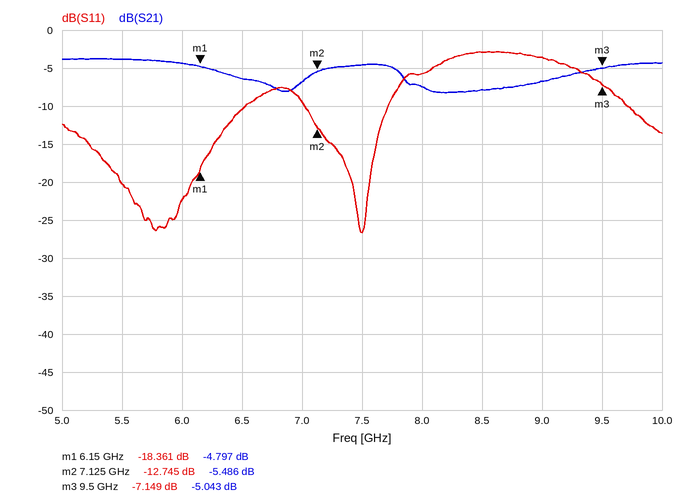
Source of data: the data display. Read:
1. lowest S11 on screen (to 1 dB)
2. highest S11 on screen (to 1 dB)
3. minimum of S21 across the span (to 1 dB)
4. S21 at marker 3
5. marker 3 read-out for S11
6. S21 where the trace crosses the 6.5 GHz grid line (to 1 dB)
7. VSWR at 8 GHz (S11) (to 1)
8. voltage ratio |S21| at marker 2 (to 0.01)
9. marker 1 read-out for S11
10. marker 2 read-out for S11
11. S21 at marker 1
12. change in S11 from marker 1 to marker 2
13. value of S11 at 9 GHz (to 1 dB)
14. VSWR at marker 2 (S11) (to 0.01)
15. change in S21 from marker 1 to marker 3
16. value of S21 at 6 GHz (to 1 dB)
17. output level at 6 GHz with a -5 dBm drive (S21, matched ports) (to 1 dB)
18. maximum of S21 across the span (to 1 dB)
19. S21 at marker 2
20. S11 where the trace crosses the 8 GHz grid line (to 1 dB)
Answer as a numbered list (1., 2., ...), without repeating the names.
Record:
1. -27 dB
2. -3 dB
3. -8 dB
4. -5.043 dB
5. -7.149 dB
6. -6 dB
7. 3
8. 0.53
9. -18.361 dB
10. -12.745 dB
11. -4.797 dB
12. 5.616 dB
13. -4 dB
14. 1.60
15. -0.246 dB
16. -4 dB
17. -9 dBm
18. -4 dB
19. -5.486 dB
20. -6 dB
